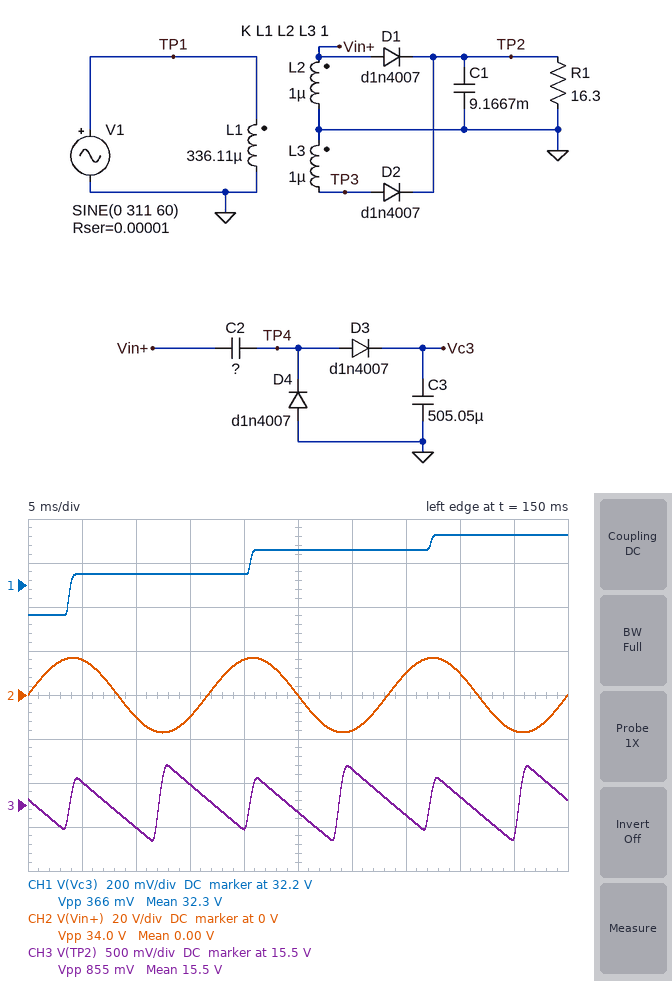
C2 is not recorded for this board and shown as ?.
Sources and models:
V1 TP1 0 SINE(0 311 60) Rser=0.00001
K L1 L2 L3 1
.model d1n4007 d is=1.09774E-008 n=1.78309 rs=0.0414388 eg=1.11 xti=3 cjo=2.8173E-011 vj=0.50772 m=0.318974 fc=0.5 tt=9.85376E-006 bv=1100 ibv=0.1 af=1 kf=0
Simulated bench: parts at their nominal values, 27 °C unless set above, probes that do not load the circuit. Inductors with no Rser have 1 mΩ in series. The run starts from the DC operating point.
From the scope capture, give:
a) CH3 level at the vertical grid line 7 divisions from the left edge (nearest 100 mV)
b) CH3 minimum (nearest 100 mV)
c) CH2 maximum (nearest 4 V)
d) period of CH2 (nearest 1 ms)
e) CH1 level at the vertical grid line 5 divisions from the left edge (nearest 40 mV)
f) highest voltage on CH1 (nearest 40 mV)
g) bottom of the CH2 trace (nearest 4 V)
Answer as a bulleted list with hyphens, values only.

- 15.4 V
- 15.1 V
- 16 V
- 17 ms
- 32.36 V
- 32.44 V
- -16 V
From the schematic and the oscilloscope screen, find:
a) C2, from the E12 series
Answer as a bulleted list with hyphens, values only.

- 330 µF
